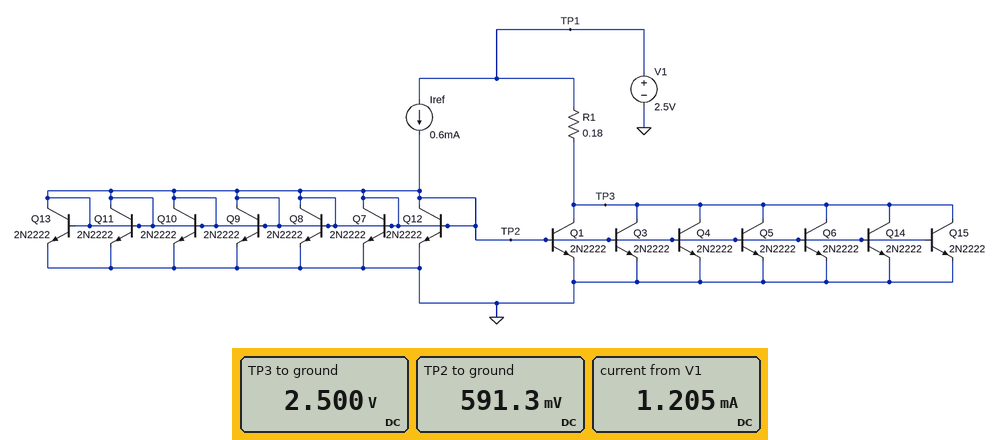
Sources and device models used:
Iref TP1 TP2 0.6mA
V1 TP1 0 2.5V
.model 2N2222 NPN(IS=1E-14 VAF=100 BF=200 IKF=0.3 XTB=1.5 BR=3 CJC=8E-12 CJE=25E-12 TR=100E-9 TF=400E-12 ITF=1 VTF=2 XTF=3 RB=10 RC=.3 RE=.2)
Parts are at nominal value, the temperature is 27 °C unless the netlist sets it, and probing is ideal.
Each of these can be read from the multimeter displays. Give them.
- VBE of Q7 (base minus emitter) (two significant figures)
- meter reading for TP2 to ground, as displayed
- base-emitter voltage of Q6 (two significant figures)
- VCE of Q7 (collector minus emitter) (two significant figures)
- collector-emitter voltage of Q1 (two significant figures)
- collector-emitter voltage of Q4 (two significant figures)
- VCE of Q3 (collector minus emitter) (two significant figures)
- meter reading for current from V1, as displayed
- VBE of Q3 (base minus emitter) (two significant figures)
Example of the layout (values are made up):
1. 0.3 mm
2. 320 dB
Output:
1. 590 mV
2. 591.3 mV
3. 590 mV
4. 590 mV
5. 2.5 V
6. 2.5 V
7. 2.5 V
8. 1.205 mA
9. 590 mV
